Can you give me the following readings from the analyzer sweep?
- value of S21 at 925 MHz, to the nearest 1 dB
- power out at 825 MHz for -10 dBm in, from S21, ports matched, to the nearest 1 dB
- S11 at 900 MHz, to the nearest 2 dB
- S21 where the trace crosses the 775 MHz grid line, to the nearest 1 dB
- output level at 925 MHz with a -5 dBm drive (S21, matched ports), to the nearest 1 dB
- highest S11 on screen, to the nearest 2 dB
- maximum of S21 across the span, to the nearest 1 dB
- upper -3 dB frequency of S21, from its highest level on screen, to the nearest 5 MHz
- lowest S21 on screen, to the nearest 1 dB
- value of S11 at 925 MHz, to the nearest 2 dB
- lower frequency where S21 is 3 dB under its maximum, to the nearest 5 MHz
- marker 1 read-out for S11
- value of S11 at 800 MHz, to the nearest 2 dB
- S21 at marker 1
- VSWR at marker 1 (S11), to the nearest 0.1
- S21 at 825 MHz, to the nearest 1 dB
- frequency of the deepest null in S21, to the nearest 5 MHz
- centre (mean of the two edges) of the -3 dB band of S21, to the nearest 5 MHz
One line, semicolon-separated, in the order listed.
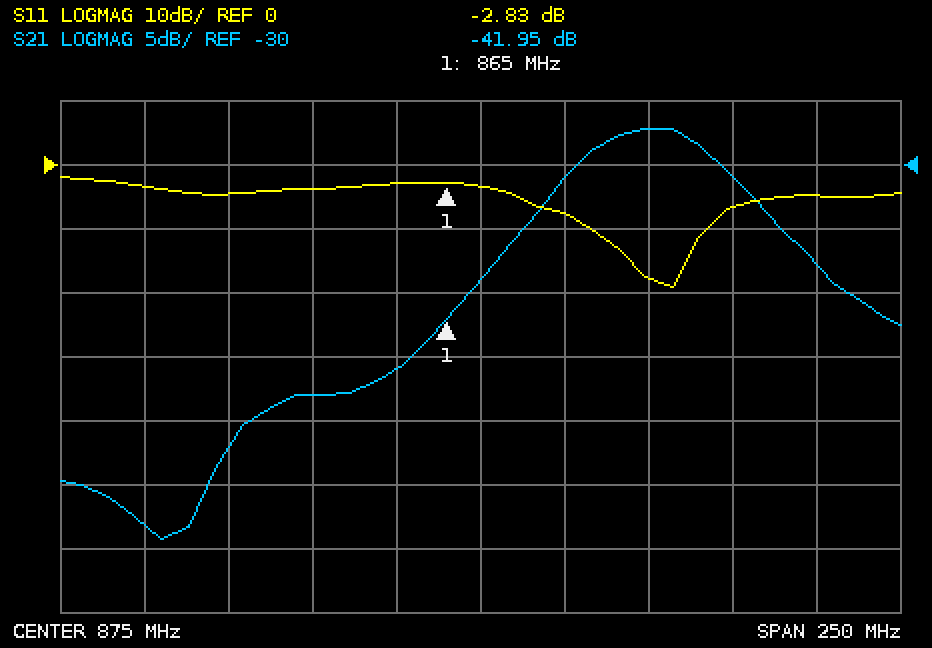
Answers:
-27 dB; -58 dBm; -8 dB; -58 dB; -32 dBm; -2 dB; -27 dB; 945 MHz; -59 dB; -18 dB; 905 MHz; -2.83 dB; -4 dB; -41.95 dB; 6.2; -48 dB; 780 MHz; 925 MHz
